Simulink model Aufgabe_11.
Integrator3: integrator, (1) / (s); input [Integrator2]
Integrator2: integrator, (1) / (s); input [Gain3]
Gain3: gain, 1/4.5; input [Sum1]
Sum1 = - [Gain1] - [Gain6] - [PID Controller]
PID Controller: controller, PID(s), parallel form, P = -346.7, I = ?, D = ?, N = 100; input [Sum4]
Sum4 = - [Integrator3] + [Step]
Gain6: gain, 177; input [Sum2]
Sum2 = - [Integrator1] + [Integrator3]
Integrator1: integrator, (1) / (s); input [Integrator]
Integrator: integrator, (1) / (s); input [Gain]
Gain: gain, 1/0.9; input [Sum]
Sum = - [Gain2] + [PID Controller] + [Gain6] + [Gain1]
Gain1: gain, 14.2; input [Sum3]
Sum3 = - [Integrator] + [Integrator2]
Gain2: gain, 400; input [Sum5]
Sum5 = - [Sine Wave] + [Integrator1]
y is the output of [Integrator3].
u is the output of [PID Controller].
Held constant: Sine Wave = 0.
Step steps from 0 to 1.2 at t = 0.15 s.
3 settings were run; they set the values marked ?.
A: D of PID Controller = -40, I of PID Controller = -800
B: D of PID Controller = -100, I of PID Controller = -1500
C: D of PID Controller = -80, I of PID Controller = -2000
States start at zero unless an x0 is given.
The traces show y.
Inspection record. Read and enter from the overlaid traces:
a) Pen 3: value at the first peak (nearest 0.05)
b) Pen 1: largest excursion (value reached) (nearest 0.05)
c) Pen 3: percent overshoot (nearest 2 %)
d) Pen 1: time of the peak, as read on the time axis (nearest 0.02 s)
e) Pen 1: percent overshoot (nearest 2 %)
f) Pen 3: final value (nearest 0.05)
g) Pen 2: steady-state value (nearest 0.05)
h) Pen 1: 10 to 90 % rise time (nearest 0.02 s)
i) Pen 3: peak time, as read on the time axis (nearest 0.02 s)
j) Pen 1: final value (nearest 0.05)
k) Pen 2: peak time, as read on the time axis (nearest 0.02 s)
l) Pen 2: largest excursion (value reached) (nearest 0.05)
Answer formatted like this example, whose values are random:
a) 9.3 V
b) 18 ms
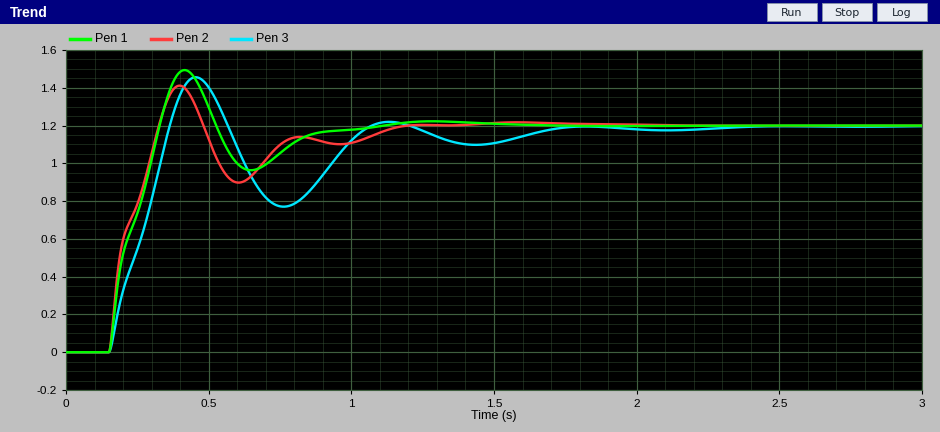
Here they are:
a) 1.45
b) 1.50
c) 22 %
d) 0.42 s
e) 24 %
f) 1.20
g) 1.20
h) 0.14 s
i) 0.46 s
j) 1.20
k) 0.40 s
l) 1.40
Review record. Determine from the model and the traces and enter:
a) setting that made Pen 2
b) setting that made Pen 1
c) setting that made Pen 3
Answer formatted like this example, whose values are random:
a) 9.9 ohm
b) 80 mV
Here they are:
a) B
b) C
c) A
